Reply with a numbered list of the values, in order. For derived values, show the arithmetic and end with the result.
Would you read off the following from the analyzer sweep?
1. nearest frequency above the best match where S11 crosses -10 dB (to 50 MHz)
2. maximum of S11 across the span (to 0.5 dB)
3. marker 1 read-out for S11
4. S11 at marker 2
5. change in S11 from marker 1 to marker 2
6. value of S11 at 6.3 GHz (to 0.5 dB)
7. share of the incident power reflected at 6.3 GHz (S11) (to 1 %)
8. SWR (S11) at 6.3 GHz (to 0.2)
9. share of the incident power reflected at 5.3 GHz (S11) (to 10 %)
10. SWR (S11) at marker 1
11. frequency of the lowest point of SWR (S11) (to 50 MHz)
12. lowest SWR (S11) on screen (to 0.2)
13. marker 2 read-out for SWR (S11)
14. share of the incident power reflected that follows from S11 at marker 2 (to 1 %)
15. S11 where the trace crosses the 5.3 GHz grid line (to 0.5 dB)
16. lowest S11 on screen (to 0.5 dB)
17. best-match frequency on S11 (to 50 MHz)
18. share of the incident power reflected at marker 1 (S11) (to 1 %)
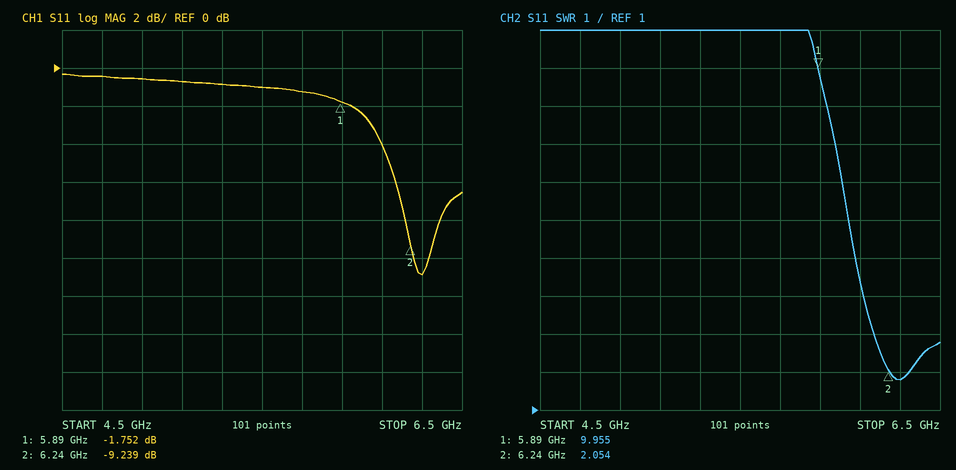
1. 6.35 GHz
2. -0.5 dB
3. -1.752 dB
4. -9.239 dB
5. -9.239 − (-1.752) = -7.487 dB
6. -11.0 dB
7. 10^(-11/10) ≈ 8 %
8. 1.8
9. 10^(-1/10) ≈ 79.4 %, so 80 % to the nearest 10 %
10. 9.955
11. 6.30 GHz
12. 1.8
13. 2.054
14. 10^(-9.239/10) ≈ 12 %
15. -1.0 dB
16. -11.0 dB
17. 6.30 GHz
18. 10^(-1.752/10) ≈ 67 %
